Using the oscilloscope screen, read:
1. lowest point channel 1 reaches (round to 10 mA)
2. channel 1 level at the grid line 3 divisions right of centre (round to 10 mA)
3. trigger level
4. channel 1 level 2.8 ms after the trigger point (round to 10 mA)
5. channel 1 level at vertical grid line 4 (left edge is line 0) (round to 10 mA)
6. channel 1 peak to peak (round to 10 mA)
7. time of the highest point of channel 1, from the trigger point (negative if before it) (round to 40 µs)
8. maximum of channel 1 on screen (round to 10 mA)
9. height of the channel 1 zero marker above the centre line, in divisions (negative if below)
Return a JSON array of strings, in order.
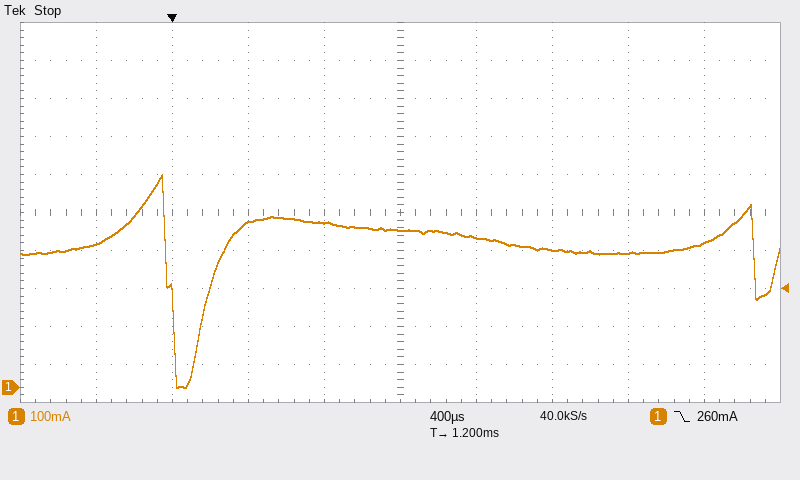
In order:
["0 mA", "350 mA", "260 mA", "380 mA", "430 mA", "560 mA", "-40 µs", "560 mA", "-4.6 div"]
